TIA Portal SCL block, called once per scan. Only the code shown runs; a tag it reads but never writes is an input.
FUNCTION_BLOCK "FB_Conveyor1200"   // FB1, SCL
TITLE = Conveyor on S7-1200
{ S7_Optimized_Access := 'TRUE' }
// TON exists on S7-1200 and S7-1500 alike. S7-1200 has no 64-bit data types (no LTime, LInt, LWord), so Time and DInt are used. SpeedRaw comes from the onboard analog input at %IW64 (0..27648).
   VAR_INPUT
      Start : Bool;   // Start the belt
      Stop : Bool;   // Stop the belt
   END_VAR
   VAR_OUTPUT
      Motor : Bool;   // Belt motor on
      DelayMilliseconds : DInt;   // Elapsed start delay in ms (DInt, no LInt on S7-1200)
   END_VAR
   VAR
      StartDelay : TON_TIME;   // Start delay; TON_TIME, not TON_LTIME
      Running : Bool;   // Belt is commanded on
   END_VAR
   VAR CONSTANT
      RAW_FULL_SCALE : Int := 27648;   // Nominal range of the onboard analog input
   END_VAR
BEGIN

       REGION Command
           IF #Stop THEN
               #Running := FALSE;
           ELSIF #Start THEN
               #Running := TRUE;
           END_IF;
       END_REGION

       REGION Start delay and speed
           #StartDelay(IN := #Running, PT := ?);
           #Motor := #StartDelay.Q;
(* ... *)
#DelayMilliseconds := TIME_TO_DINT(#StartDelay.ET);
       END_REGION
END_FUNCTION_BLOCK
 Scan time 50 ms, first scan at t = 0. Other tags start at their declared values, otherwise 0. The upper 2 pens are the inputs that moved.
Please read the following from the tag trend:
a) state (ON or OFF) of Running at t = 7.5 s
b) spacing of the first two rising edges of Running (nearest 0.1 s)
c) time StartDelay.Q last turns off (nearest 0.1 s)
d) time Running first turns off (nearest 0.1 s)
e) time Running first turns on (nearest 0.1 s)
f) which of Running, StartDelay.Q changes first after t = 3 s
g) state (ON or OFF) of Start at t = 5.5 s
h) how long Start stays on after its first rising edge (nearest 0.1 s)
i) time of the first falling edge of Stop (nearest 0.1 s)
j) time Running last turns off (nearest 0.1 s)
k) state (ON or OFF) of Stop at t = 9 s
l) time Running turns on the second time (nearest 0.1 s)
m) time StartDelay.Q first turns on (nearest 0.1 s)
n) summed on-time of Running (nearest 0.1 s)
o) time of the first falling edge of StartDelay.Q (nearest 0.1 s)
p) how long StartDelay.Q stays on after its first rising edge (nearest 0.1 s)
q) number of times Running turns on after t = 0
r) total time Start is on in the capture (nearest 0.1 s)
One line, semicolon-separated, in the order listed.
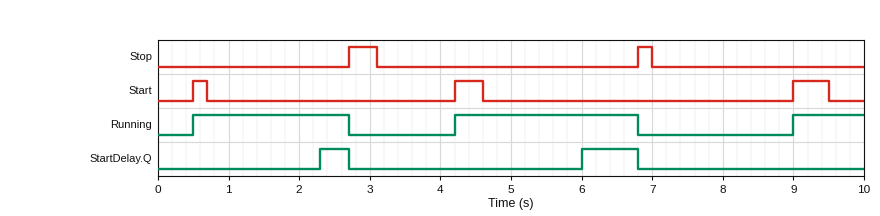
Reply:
OFF; 3.7 s; 6.8 s; 2.7 s; 0.5 s; Running; OFF; 0.2 s; 3.1 s; 6.8 s; OFF; 4.2 s; 2.3 s; 5.8 s; 2.7 s; 0.4 s; 3; 1.1 s
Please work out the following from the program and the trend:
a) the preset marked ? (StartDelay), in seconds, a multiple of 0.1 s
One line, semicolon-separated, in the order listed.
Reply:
1.8 s
